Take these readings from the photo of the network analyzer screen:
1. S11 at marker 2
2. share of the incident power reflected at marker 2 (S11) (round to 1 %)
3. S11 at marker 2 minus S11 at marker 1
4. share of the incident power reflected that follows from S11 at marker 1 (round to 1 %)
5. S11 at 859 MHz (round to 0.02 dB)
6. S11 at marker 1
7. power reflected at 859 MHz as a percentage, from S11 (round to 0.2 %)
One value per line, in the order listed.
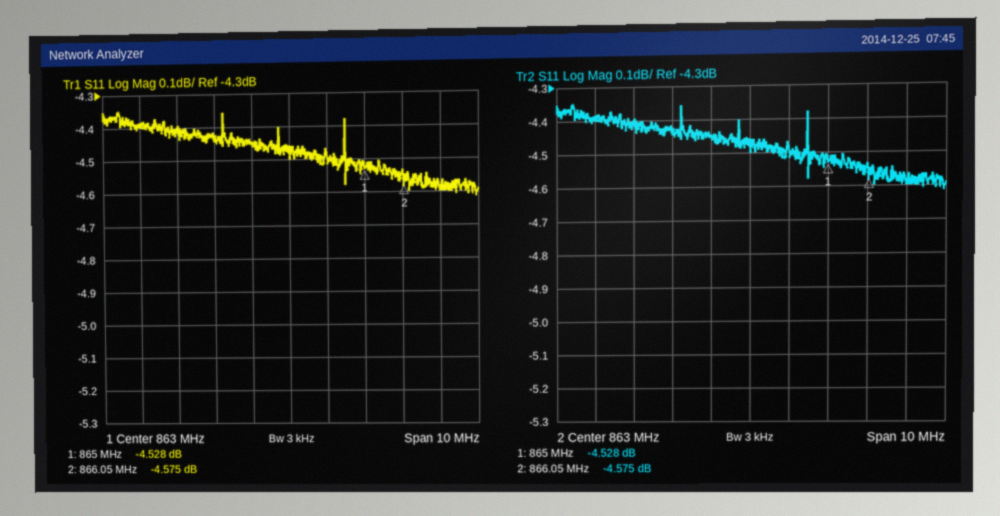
-4.575 dB
35 %
-0.047 dB
35 %
-4.40 dB
-4.528 dB
36.4 %
